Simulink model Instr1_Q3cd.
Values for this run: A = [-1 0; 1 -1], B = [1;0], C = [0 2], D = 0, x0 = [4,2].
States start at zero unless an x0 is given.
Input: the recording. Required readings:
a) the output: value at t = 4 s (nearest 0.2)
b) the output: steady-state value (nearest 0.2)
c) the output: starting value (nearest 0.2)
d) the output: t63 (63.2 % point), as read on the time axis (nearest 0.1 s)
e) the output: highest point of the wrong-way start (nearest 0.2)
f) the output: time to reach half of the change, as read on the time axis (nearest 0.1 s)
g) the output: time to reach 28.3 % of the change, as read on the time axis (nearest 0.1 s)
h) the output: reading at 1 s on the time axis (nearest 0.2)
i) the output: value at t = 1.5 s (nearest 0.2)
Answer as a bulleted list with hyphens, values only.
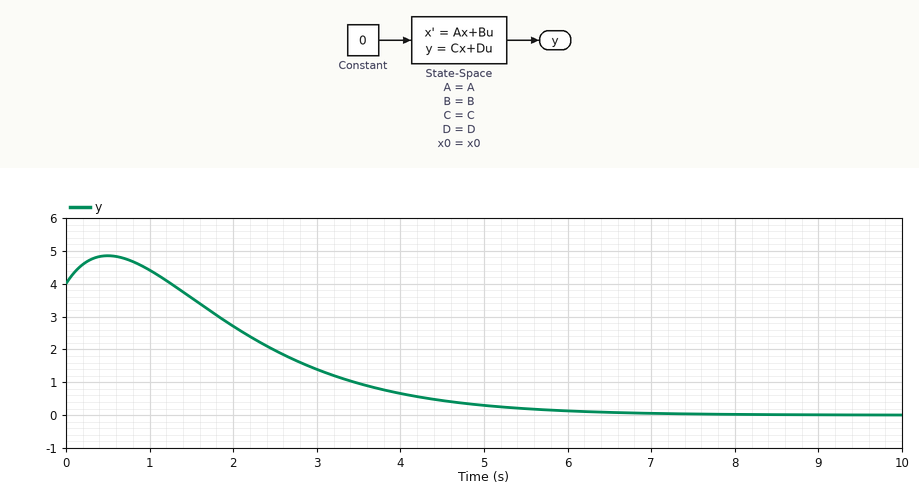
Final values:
- 0.6
- 0.0
- 4.0
- 2.9 s
- 4.8
- 2.5 s
- 1.9 s
- 4.4
- 3.6
